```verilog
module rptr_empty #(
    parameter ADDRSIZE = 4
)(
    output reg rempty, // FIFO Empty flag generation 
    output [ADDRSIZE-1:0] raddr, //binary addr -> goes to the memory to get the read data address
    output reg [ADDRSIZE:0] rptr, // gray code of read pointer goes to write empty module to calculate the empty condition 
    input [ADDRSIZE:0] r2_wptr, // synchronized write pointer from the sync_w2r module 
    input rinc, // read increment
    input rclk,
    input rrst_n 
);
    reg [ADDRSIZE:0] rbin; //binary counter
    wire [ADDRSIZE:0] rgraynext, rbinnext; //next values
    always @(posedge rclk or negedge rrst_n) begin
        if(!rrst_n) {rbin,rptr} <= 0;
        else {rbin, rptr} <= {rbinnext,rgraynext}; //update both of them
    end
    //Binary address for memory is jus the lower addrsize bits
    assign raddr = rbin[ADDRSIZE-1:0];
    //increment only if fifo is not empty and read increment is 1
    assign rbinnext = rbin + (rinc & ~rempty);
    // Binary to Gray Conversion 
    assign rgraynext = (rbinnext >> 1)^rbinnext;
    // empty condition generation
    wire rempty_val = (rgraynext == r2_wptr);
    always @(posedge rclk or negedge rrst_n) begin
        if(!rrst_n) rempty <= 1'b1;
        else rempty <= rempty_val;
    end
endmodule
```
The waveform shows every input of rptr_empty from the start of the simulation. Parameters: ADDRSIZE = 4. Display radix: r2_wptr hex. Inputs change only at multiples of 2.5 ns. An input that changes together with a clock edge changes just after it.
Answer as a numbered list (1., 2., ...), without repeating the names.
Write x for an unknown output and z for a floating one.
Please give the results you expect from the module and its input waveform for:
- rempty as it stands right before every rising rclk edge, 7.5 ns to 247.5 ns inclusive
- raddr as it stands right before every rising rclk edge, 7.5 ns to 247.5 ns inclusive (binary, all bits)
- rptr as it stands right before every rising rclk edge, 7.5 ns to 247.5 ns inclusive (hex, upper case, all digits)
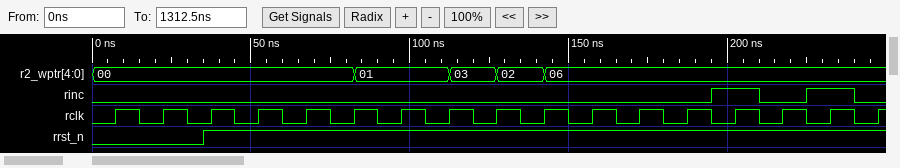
1. 1 1 1 1 1 1 1 0 0 0 0 0 0 0 0 0 0
2. 0000, 0000, 0000, 0000, 0000, 0000, 0000, 0000, 0000, 0000, 0000, 0000, 0000, 0000, 0001, 0001, 0010
3. 00, 00, 00, 00, 00, 00, 00, 00, 00, 00, 00, 00, 00, 00, 01, 01, 03
